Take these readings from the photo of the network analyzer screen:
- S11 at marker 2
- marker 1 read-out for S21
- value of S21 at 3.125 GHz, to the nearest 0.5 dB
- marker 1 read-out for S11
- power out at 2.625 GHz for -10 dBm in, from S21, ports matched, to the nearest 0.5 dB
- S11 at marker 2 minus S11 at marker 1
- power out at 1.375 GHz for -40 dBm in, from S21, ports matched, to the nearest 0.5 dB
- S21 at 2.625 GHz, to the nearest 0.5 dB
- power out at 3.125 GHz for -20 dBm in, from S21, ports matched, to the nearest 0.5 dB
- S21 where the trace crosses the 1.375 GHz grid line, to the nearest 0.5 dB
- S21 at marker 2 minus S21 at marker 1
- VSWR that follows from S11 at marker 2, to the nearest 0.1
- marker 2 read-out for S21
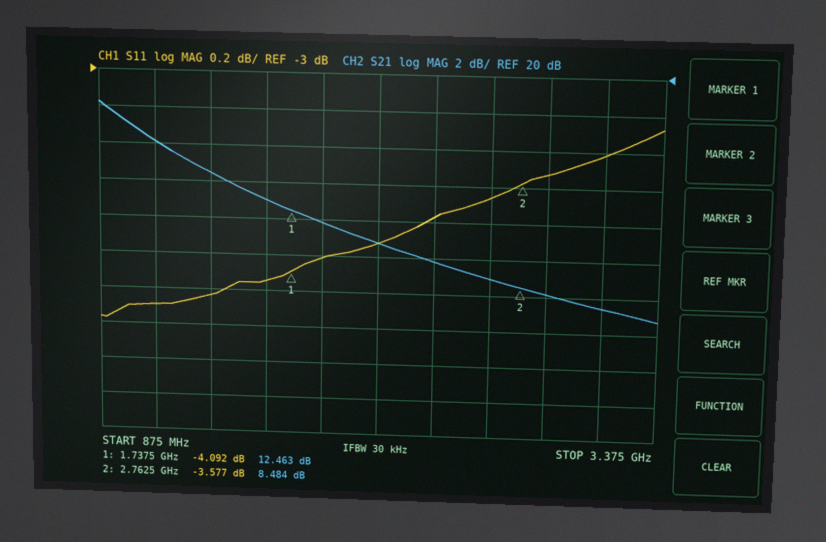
-3.577 dB
12.463 dB
7.5 dB
-4.092 dB
-1.0 dBm
0.515 dB
-25.5 dBm
9.0 dB
-12.5 dBm
14.5 dB
-3.979 dB
4.9
8.484 dB
